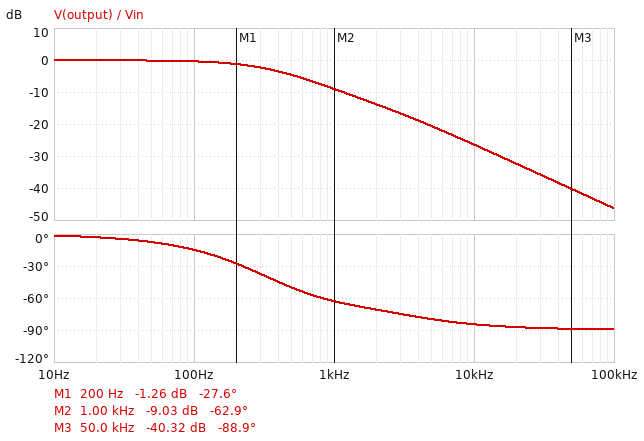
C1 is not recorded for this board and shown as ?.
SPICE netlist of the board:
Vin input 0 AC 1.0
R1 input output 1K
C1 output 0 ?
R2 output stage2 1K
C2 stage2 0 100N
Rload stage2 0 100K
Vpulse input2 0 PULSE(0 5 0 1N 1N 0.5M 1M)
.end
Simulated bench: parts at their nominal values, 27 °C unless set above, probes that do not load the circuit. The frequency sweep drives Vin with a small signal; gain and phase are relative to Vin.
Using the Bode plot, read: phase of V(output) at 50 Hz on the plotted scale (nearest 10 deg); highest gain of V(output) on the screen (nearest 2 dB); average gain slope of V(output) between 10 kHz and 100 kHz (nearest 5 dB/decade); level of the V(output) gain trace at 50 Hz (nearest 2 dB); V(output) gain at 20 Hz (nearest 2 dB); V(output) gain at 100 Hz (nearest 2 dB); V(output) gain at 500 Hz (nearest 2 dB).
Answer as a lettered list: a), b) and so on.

a) -10 deg
b) 0 dB
c) -20 dB/decade
d) 0 dB
e) 0 dB
f) 0 dB
g) -4 dB
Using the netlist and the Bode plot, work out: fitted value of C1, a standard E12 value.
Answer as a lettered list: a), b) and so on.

a) 330 nF
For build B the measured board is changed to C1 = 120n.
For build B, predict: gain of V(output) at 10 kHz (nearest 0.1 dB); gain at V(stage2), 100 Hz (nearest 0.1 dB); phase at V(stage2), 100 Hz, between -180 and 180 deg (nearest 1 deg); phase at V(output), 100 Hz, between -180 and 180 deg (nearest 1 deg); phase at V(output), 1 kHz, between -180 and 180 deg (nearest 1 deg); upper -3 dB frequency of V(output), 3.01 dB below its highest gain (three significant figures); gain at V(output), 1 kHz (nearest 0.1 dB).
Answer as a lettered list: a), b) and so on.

a) -18.0 dB
b) -0.3 dB
c) -11 deg
d) -8 deg
e) -43 deg
f) 659 Hz
g) -4.9 dB
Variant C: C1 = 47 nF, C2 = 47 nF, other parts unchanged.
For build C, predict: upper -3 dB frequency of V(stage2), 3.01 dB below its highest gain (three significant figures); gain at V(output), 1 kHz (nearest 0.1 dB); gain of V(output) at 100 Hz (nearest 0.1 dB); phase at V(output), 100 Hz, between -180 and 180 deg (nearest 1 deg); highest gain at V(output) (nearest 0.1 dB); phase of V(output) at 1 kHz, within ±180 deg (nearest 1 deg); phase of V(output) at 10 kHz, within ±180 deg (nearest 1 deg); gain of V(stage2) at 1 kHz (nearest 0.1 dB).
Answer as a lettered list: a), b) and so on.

a) 1.29 kHz
b) -1.8 dB
c) -0.1 dB
d) -3 deg
e) -0.1 dB
f) -27 deg
g) -60 deg
h) -2.2 dB
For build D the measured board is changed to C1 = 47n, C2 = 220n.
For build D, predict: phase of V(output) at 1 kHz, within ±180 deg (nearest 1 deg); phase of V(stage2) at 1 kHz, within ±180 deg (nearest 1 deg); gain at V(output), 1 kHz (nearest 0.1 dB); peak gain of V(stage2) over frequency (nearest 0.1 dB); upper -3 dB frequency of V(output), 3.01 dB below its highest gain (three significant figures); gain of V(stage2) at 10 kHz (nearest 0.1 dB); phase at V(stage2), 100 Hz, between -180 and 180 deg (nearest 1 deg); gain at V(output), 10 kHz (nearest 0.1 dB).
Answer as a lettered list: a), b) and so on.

a) -25 deg
b) -79 deg
c) -5.2 dB
d) -0.2 dB
e) 471 Hz
f) -34.0 dB
g) -17 deg
h) -11.2 dB
